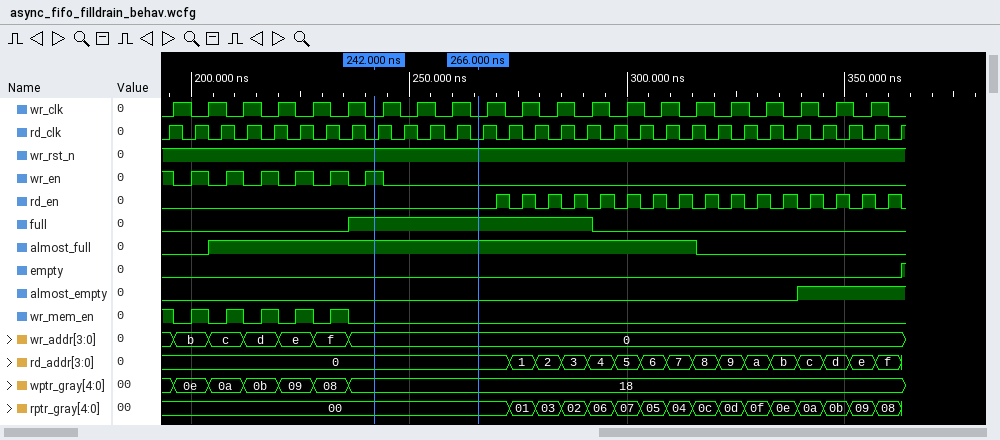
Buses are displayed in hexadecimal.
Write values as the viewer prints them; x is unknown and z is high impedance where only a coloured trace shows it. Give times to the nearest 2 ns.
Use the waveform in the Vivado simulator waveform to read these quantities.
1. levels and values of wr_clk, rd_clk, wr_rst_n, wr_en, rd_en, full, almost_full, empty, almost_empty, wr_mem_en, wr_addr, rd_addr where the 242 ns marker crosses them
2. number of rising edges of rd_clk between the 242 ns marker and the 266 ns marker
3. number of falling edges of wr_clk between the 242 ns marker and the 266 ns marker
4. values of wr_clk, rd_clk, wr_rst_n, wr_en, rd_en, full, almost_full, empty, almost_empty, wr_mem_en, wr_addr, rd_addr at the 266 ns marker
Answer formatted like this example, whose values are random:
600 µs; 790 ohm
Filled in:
wr_clk=0, rd_clk=0, wr_rst_n=1, wr_en=1, rd_en=0, full=1, almost_full=1, empty=0, almost_empty=0, wr_mem_en=0, wr_addr=0, rd_addr=0; 4; 3; wr_clk=0, rd_clk=0, wr_rst_n=1, wr_en=0, rd_en=0, full=1, almost_full=1, empty=0, almost_empty=0, wr_mem_en=0, wr_addr=0, rd_addr=0
